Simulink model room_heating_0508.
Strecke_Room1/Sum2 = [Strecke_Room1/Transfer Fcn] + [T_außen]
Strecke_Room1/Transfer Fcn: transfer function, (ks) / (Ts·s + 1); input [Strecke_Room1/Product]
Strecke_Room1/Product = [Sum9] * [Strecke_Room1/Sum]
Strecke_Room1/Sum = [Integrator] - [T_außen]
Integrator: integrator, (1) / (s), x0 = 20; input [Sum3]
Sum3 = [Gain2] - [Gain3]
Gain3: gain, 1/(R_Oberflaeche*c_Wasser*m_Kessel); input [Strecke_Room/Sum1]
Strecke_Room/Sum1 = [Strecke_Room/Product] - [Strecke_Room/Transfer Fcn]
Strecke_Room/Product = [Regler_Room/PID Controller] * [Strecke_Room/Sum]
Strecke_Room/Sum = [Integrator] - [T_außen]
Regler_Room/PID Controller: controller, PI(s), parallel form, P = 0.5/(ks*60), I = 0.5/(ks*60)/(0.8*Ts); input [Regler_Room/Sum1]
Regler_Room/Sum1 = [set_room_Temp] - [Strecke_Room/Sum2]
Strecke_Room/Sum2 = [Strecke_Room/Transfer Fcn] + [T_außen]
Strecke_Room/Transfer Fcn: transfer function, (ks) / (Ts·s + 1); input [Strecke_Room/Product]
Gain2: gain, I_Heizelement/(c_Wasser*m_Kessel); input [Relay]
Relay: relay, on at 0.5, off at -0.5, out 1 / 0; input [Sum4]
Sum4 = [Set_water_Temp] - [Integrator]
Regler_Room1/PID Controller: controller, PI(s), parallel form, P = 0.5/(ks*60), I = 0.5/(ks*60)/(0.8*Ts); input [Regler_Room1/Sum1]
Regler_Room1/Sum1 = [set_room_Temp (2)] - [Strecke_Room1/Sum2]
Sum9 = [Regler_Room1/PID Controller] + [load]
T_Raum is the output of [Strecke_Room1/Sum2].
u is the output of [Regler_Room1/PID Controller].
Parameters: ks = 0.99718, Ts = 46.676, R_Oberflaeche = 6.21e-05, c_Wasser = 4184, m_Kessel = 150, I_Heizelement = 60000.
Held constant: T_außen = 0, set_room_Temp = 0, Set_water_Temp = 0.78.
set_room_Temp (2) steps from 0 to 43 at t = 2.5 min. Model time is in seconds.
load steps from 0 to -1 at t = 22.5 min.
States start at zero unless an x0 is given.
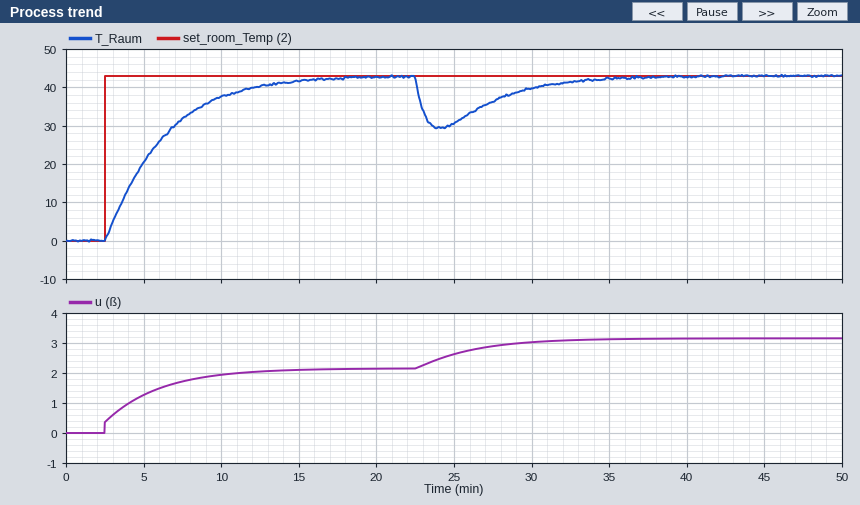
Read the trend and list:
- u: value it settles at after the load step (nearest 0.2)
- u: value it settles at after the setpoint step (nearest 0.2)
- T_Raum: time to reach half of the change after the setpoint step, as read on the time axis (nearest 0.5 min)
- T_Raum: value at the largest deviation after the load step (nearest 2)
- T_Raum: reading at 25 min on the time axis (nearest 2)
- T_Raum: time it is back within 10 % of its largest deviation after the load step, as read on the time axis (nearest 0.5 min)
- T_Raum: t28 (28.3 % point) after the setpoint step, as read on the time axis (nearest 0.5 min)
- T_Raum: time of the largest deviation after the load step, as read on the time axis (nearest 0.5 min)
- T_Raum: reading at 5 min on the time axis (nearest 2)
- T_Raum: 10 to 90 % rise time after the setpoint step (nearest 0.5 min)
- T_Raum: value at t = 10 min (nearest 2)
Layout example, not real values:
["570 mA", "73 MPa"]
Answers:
["3.2", "2.2", "5.0 min", "30", "30", "33.0 min", "4.0 min", "24.0 min", "20", "8.0 min", "38"]
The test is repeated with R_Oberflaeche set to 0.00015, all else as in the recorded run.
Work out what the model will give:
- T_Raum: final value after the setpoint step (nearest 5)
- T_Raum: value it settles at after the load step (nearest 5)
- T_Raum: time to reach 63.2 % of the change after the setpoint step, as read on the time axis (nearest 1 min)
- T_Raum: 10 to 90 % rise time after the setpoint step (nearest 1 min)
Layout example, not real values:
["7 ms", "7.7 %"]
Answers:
["45", "45", "6 min", "8 min"]
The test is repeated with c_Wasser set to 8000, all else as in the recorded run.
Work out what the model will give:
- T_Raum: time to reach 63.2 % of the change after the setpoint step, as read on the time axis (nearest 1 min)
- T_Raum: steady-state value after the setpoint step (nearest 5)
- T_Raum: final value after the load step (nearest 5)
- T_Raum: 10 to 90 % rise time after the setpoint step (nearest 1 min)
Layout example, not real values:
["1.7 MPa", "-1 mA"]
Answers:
["6 min", "45", "45", "8 min"]
